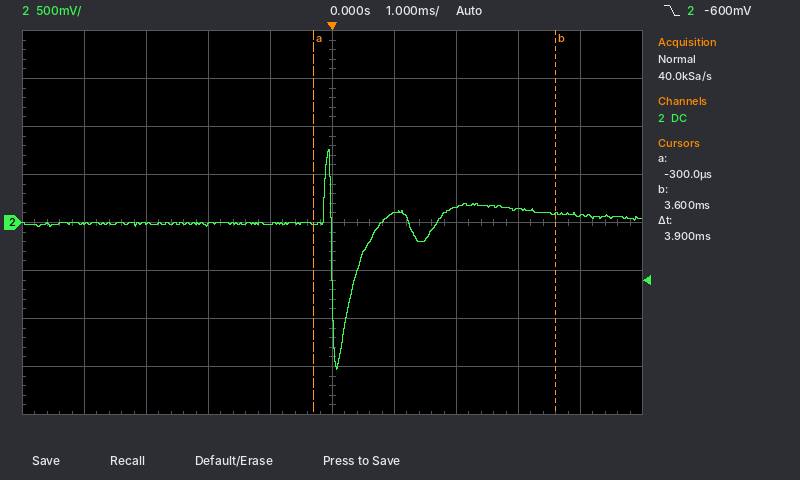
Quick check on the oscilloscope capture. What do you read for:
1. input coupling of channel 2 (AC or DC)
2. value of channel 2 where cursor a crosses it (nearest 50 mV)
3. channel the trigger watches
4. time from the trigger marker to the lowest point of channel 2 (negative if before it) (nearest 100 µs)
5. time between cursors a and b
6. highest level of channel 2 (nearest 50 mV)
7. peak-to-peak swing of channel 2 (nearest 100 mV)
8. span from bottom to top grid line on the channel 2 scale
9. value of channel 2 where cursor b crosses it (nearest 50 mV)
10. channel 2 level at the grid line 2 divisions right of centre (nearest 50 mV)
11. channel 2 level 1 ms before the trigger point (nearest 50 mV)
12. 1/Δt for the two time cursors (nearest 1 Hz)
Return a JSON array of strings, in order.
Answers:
["DC", "0 mV", "channel 2", "+100 µs", "3.9 ms", "750 mV", "2.30 V", "4 V", "100 mV", "150 mV", "0 mV", "256 Hz"]
